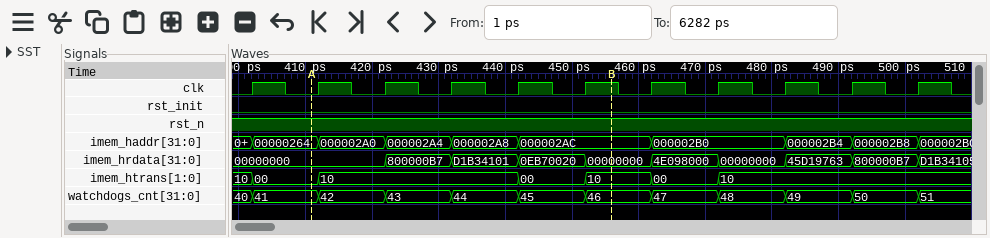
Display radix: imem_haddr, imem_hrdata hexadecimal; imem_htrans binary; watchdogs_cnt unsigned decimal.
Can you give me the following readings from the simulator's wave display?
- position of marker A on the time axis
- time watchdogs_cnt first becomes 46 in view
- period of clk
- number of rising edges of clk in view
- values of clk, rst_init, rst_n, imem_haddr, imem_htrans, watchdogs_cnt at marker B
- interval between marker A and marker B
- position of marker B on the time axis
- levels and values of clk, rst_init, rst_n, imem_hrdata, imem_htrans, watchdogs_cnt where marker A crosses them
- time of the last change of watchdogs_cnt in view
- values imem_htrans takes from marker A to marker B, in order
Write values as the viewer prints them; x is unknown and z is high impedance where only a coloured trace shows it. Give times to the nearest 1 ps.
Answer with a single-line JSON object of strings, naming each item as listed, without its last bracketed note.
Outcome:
{"position of marker A on the time axis": "411 ps", "time watchdogs_cnt first becomes 46 in view": "452 ps", "period of clk": "10 ps", "number of rising edges of clk in view": "11", "values of clk, rst_init, rst_n, imem_haddr, imem_htrans, watchdogs_cnt at marker B": "clk=1, rst_init=0, rst_n=1, imem_haddr=000002AC, imem_htrans=10, watchdogs_cnt=46", "interval between marker A and marker B": "45 ps", "position of marker B on the time axis": "456 ps", "levels and values of clk, rst_init, rst_n, imem_hrdata, imem_htrans, watchdogs_cnt where marker A crosses them": "clk=0, rst_init=0, rst_n=1, imem_hrdata=00000000, imem_htrans=00, watchdogs_cnt=41", "time of the last change of watchdogs_cnt in view": "502 ps", "values imem_htrans takes from marker A to marker B, in order": "00, 10, 00, 10"}
